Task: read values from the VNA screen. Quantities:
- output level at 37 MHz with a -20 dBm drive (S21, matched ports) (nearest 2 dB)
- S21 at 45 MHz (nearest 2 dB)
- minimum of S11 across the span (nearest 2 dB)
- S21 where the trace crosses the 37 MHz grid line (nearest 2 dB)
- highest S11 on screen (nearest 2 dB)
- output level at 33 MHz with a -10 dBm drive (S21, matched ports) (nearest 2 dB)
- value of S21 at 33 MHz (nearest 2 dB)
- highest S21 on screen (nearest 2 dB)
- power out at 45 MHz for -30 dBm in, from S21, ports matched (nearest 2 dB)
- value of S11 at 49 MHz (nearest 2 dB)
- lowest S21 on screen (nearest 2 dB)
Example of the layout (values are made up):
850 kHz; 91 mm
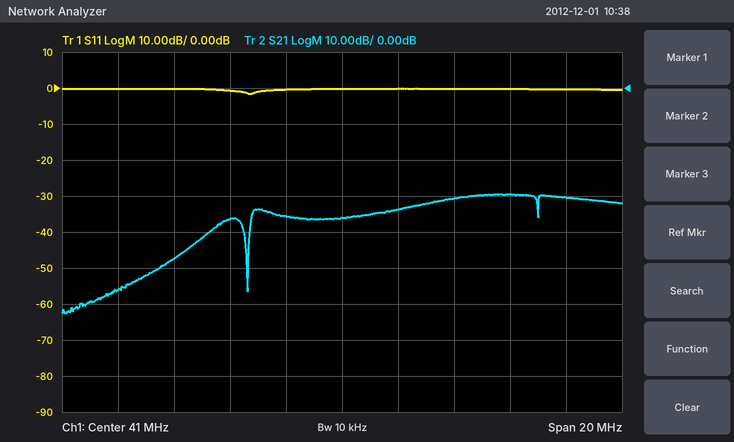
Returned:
-56 dBm; -30 dB; -2 dB; -36 dB; 0 dB; -66 dBm; -56 dB; -30 dB; -60 dBm; 0 dB; -62 dB
